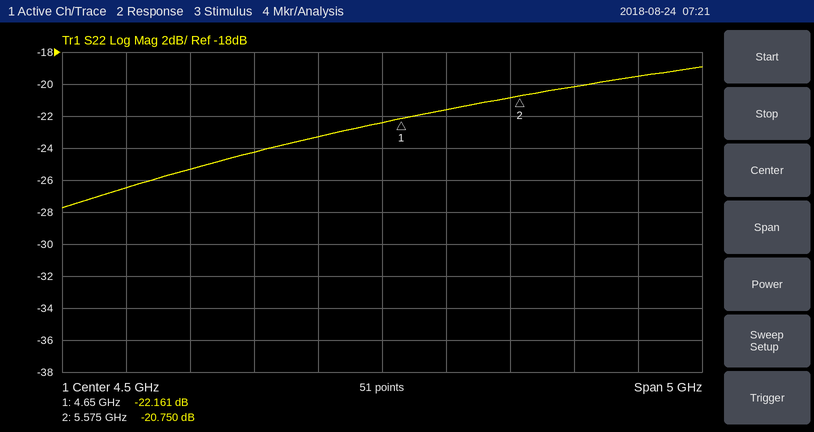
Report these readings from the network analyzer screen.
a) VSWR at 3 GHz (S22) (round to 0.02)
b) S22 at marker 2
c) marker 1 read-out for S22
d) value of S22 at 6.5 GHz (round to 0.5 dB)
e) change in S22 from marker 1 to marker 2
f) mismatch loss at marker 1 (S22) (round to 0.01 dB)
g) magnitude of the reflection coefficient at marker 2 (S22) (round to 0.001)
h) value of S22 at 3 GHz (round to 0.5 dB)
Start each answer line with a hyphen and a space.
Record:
- 1.12
- -20.750 dB
- -22.161 dB
- -19.5 dB
- 1.411 dB
- 0.03 dB
- 0.092
- -25.5 dB
